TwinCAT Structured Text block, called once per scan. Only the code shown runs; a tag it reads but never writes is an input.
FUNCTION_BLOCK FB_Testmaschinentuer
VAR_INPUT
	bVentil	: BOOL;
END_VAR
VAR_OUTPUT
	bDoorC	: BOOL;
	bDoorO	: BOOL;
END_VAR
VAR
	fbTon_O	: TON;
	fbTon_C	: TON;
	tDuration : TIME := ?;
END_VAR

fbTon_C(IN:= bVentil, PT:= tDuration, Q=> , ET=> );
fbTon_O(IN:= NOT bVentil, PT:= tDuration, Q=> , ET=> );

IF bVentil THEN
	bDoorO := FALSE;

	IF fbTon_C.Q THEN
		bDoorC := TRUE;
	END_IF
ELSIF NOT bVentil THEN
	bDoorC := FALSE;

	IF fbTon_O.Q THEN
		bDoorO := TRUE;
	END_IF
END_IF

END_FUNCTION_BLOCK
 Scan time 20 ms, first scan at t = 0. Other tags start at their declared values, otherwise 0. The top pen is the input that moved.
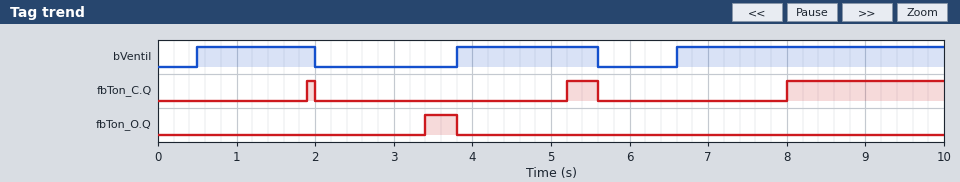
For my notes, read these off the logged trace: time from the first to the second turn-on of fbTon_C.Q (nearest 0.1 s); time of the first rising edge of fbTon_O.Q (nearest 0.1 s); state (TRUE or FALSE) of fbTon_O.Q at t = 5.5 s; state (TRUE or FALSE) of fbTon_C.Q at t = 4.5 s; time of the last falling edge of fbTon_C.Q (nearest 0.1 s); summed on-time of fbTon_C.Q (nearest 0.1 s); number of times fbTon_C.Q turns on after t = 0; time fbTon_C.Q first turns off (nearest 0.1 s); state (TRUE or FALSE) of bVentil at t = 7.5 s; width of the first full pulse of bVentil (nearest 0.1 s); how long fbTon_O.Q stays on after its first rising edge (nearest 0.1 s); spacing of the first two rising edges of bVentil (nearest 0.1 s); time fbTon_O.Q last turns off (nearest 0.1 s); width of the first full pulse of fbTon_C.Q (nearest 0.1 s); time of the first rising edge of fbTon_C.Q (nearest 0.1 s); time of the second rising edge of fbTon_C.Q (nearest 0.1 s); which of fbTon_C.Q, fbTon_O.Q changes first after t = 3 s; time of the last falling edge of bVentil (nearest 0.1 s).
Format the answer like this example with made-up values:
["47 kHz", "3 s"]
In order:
["3.3 s", "3.4 s", "FALSE", "FALSE", "5.6 s", "2.5 s", "3", "2.0 s", "TRUE", "1.5 s", "0.4 s", "3.3 s", "3.8 s", "0.1 s", "1.9 s", "5.2 s", "fbTon_O.Q", "5.6 s"]
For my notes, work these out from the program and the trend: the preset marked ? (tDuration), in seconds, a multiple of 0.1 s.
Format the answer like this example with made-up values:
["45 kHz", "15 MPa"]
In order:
["1.4 s"]
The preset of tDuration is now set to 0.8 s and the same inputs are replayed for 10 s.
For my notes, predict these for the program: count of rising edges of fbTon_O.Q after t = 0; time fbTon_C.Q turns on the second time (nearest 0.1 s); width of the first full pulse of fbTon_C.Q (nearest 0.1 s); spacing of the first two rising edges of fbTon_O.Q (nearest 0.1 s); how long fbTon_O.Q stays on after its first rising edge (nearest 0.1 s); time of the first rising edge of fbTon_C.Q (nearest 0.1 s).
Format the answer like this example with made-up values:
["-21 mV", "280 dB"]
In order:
["2", "4.6 s", "0.7 s", "3.6 s", "1.0 s", "1.3 s"]
